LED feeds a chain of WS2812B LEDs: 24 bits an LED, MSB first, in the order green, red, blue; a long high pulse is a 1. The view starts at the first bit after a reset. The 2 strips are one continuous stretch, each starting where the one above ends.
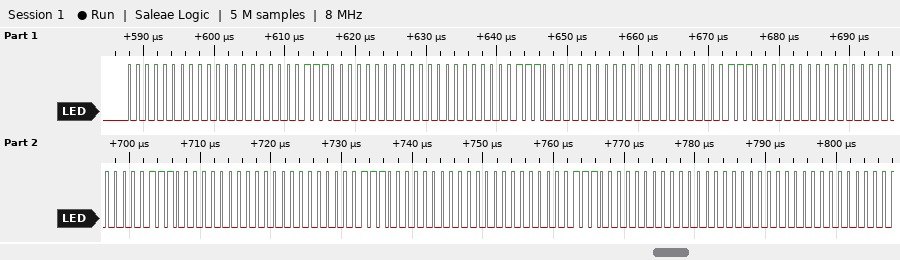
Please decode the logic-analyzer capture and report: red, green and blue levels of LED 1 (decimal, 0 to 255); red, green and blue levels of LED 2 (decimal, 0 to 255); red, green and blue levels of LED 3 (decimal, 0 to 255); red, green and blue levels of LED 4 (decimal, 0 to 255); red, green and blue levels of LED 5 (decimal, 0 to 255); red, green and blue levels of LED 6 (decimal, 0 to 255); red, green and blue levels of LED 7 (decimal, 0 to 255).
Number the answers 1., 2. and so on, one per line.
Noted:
1. 0, 0, 14
2. 0, 0, 14
3. 0, 0, 14
4. 0, 0, 14
5. 0, 0, 14
6. 0, 0, 14
7. 0, 0, 0
